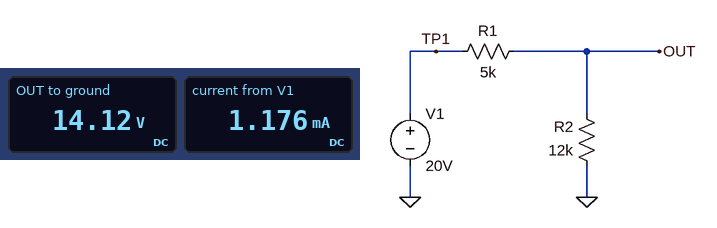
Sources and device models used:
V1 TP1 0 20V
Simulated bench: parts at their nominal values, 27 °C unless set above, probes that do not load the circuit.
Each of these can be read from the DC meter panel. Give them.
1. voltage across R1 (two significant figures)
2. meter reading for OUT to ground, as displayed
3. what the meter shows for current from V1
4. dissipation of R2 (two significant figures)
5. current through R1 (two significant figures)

5.9 V
14.12 V
1.176 mA
17 mW
1.2 mA
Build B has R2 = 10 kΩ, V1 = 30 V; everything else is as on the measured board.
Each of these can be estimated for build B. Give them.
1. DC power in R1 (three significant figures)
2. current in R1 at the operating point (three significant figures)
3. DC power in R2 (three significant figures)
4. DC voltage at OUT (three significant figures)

20.0 mW
2.00 mA
40.0 mW
20.0 V
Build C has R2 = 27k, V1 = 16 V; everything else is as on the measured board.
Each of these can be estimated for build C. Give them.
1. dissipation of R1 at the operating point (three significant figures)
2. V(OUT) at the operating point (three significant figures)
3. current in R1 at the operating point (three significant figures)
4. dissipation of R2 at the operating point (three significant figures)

1.25 mW
13.5 V
500 µA
6.75 mW
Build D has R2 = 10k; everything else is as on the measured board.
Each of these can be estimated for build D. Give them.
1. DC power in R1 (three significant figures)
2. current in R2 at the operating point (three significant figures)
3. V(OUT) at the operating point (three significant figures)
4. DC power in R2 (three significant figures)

8.89 mW
1.33 mA
13.3 V
17.8 mW
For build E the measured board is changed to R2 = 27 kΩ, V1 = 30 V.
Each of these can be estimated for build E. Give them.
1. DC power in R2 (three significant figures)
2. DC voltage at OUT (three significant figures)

23.7 mW
25.3 V
